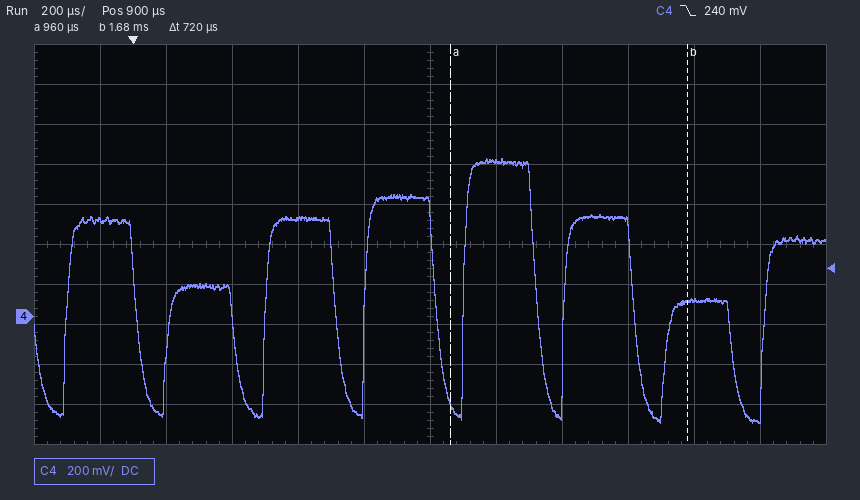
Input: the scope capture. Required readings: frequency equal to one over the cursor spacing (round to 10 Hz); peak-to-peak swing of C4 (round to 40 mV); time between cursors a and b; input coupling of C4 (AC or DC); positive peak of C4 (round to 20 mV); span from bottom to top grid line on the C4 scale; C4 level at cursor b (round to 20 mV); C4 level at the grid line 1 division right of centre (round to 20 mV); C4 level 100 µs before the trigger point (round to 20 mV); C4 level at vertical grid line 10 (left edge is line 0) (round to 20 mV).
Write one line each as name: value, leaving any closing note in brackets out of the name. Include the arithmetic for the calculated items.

frequency equal to one over the cursor spacing: 1 / 720 µs ≈ 1.39 kHz
peak-to-peak swing of C4: 1.32 V
time between cursors a and b: 720 µs
input coupling of C4: DC
positive peak of C4: 800 mV
span from bottom to top grid line on the C4 scale: 2 V
C4 level at cursor b: 80 mV
C4 level at the grid line 1 division right of centre: 780 mV
C4 level 100 µs before the trigger point: 480 mV
C4 level at vertical grid line 10 (left edge is line 0): 80 mV
